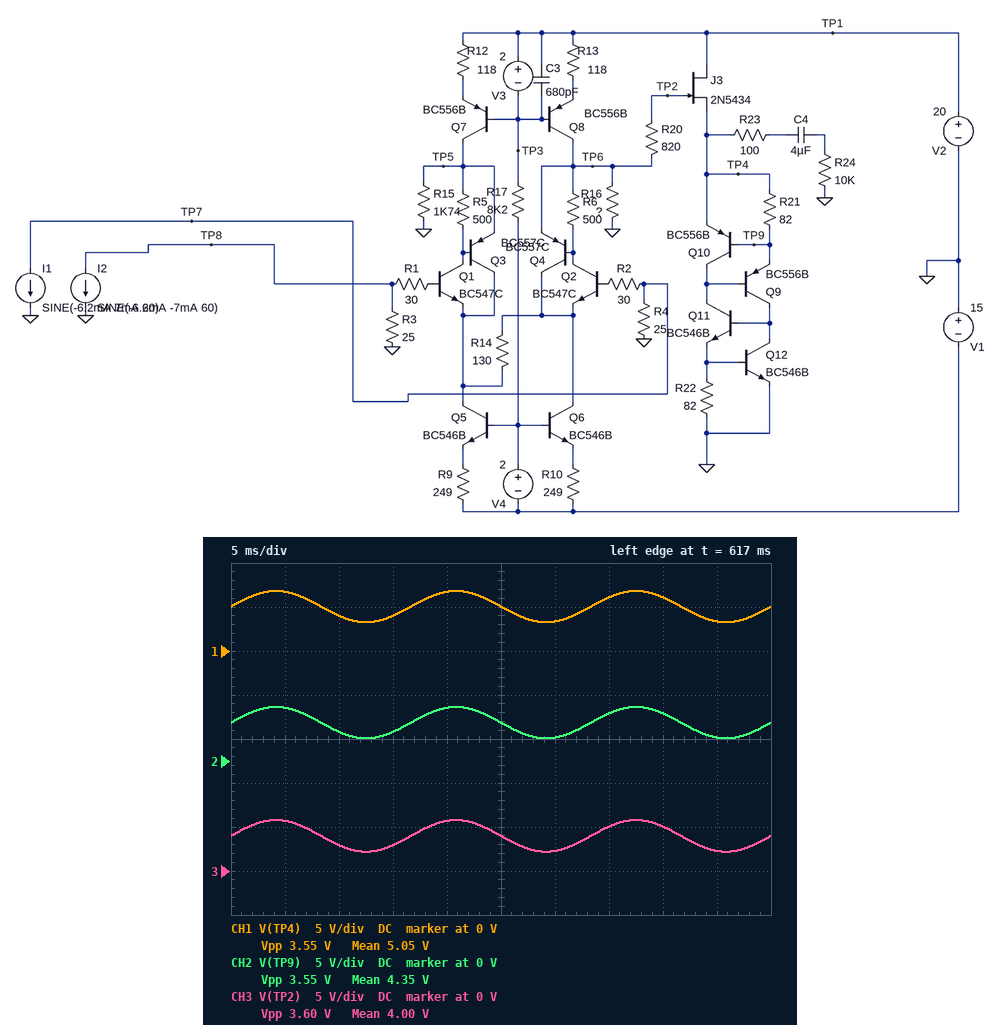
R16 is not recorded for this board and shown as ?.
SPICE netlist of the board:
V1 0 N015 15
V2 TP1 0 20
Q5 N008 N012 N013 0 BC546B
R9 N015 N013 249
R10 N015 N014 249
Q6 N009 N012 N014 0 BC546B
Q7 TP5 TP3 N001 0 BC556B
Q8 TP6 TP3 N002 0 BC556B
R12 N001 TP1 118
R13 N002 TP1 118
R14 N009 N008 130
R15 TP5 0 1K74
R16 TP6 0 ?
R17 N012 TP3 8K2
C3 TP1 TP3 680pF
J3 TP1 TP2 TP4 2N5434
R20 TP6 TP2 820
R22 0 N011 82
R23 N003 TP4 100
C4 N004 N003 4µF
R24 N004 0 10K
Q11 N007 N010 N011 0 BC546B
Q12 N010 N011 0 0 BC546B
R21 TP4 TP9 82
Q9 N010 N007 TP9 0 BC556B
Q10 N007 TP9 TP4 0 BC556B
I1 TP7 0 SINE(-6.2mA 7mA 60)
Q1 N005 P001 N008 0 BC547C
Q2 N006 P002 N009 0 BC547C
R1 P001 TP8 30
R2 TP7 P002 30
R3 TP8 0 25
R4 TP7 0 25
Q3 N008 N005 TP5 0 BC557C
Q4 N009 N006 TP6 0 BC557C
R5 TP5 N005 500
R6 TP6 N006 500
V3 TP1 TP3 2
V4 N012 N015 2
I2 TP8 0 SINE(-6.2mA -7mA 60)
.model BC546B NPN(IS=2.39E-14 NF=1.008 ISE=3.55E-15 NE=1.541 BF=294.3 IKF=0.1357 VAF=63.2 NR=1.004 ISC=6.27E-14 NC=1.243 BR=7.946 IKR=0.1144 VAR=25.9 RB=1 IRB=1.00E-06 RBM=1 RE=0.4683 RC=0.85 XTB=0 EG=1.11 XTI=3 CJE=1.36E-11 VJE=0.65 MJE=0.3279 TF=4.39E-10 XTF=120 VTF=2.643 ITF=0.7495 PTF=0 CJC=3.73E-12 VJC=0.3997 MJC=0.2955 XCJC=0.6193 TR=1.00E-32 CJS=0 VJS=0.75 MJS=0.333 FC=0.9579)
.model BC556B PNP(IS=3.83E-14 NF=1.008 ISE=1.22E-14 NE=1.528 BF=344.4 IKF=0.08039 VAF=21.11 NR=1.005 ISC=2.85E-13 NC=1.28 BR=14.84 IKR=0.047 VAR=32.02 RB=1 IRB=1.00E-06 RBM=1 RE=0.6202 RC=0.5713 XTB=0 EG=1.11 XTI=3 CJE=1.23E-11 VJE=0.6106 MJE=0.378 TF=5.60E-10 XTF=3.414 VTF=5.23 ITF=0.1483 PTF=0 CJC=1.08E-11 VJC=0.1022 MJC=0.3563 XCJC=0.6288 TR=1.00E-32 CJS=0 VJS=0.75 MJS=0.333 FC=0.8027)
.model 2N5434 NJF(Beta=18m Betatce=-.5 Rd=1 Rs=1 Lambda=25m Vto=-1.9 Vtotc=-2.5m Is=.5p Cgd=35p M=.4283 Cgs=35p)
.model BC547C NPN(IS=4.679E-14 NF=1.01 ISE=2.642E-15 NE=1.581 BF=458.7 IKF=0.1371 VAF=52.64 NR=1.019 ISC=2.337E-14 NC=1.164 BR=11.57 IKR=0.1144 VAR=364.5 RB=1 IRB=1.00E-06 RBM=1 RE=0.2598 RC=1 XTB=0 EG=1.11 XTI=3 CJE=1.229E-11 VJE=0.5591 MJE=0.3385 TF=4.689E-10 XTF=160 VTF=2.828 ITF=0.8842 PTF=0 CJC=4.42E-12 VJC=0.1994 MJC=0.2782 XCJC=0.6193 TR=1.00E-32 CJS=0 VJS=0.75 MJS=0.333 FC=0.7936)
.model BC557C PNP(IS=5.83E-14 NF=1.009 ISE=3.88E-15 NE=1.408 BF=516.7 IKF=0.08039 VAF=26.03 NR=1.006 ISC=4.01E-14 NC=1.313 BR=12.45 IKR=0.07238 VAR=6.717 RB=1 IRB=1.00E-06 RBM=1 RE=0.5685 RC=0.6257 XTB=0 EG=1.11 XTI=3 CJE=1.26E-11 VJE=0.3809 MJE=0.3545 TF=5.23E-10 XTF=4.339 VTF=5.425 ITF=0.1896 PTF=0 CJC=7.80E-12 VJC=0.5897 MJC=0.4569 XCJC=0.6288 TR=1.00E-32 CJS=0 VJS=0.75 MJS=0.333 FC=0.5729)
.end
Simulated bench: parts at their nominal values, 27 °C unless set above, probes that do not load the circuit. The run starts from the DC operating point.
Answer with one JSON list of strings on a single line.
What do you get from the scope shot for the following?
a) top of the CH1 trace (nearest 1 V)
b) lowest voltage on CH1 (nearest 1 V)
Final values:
["7 V", "3 V"]
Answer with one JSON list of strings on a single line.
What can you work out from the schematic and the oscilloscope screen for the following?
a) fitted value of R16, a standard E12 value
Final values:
["680 Ω"]
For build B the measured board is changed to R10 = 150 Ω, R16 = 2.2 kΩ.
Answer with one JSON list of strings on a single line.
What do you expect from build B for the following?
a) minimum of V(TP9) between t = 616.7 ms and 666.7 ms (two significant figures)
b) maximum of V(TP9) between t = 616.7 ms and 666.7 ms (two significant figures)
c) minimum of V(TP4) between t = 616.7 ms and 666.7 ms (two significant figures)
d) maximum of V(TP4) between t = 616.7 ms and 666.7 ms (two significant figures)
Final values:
["1.3 V", "11 V", "1.8 V", "12 V"]
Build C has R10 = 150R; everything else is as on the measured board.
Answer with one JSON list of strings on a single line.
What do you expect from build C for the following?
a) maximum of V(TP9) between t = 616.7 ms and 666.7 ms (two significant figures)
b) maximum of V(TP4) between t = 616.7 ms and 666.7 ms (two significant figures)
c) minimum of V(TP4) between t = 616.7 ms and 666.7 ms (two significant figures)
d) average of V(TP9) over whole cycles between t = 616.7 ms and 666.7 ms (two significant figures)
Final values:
["3.9 V", "4.6 V", "1.8 V", "2.3 V"]
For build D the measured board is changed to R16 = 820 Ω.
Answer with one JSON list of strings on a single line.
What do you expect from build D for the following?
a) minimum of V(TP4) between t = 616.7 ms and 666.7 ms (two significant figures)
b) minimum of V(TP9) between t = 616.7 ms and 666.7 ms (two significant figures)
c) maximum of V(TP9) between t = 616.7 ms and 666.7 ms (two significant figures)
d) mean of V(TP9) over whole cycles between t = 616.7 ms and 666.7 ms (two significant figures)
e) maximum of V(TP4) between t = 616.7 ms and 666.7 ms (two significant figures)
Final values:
["3.7 V", "3.0 V", "7.3 V", "5.2 V", "8.0 V"]
